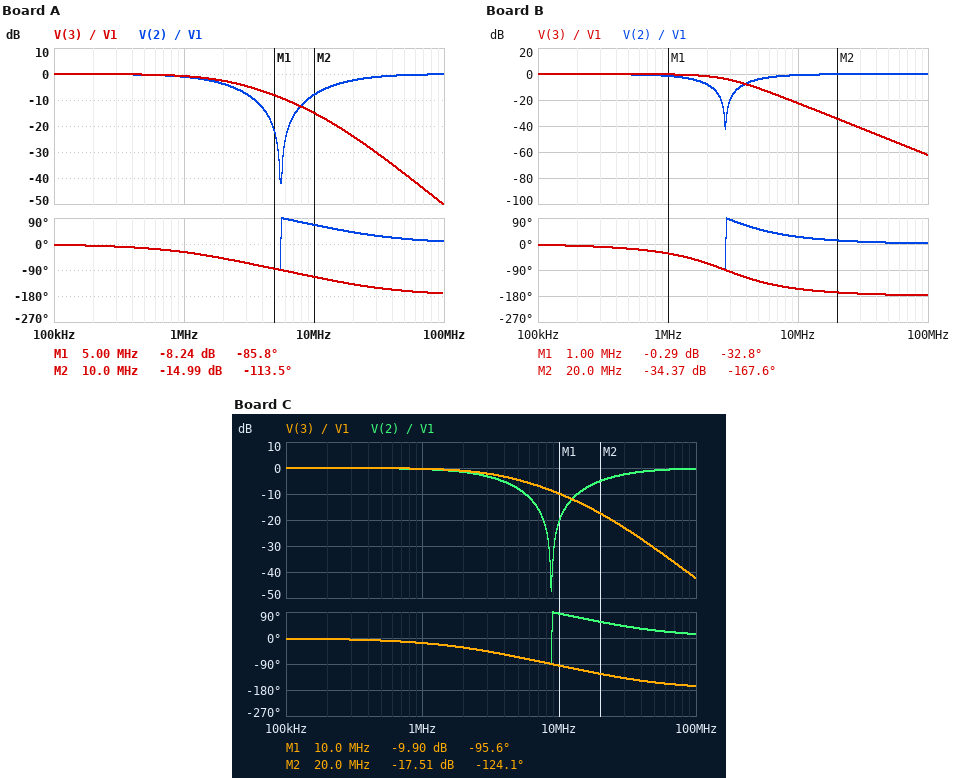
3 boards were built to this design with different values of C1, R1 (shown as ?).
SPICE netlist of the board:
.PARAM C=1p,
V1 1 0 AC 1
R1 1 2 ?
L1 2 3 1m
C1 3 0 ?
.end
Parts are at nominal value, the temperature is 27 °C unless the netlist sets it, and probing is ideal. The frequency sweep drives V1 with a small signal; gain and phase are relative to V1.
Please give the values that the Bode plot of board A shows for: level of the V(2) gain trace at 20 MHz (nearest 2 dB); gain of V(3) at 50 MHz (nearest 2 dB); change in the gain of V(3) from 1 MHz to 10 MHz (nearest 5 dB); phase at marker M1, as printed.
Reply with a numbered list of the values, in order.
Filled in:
1. -2 dB
2. -38 dB
3. -15 dB
4. -85.8 deg
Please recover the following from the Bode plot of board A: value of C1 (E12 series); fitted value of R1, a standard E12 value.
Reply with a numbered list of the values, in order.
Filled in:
1. 820 fF
2. 100 kΩ
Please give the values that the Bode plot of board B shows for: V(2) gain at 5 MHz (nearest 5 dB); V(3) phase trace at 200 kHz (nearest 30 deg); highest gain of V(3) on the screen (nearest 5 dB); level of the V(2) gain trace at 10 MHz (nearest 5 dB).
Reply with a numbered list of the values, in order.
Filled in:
1. -5 dB
2. 0 deg
3. 0 dB
4. 0 dB
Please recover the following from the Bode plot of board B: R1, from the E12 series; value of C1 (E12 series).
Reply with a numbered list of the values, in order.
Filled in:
1. 27 kΩ
2. 3.3 pF
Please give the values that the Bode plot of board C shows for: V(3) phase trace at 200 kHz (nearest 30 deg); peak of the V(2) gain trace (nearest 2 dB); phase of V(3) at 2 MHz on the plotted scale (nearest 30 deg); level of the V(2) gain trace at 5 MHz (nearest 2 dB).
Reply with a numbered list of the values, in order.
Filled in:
1. 0 deg
2. 0 dB
3. -30 deg
4. -8 dB
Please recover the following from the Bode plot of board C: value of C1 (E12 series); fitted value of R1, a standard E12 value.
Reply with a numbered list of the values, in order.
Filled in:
1. 330 fF
2. 150 kΩ
